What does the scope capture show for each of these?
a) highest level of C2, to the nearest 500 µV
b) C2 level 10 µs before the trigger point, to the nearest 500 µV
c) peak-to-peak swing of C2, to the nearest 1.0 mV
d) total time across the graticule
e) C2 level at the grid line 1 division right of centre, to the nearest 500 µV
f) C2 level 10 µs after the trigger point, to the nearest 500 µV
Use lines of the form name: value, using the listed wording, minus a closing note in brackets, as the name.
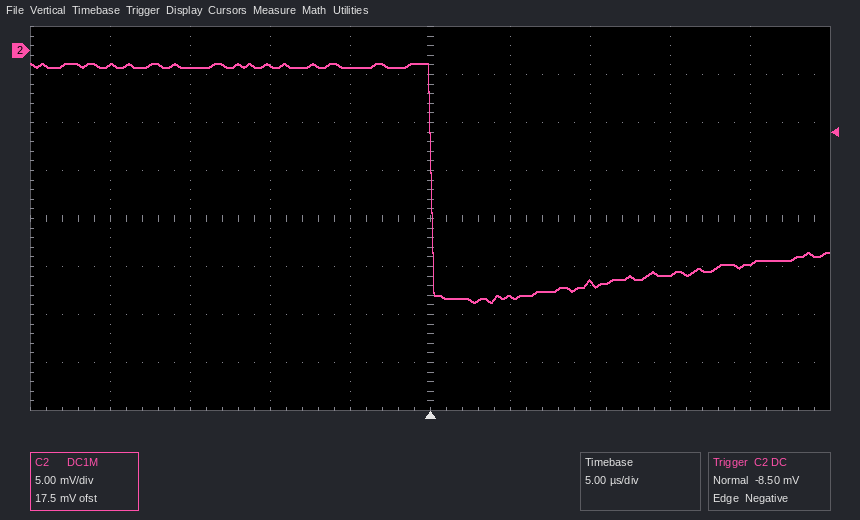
highest level of C2, to the nearest 500 µV: -1.5 mV
C2 level 10 µs before the trigger point, to the nearest 500 µV: -1.5 mV
peak-to-peak swing of C2, to the nearest 1.0 mV: 25.0 mV
total time across the graticule: 50 µs
C2 level at the grid line 1 division right of centre, to the nearest 500 µV: -25.5 mV
C2 level 10 µs after the trigger point, to the nearest 500 µV: -24.0 mV
